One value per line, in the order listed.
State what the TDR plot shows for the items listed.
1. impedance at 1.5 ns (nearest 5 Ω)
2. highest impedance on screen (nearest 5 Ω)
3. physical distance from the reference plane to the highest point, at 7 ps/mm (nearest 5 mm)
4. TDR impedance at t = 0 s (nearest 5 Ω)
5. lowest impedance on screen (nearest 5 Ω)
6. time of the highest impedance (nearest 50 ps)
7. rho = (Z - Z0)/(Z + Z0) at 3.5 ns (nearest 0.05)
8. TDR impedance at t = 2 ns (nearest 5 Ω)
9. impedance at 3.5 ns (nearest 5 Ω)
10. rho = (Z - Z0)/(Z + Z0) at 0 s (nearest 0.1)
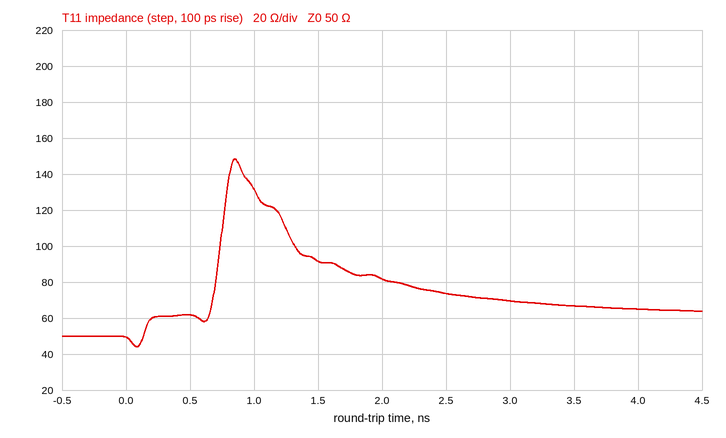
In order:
90 Ω
150 Ω
60 mm
50 Ω
45 Ω
850 ps
+0.15
80 Ω
65 Ω
0.0
